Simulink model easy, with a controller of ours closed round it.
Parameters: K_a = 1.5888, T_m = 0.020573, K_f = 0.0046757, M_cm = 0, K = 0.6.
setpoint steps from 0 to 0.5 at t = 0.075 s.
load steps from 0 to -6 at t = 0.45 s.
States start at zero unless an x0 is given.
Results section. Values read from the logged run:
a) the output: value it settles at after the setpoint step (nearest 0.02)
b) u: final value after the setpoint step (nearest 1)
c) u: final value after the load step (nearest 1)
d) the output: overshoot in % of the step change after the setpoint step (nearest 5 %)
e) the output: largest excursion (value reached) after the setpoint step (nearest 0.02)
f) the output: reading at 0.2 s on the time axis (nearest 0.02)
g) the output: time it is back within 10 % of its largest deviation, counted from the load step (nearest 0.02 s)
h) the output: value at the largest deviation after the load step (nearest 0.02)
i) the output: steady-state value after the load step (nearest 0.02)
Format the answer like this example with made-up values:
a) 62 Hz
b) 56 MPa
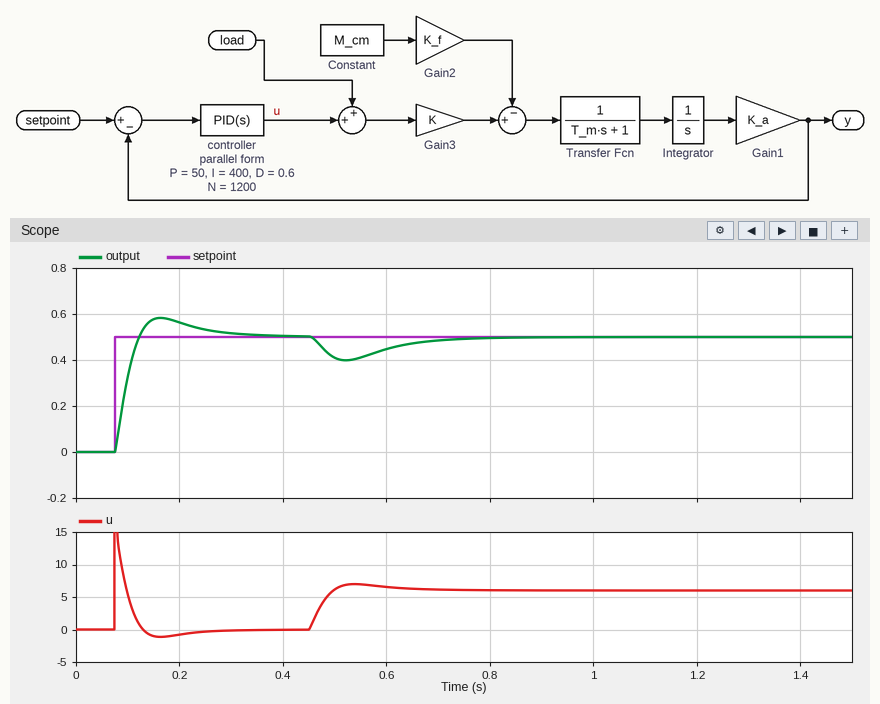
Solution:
a) 0.50
b) 0
c) 6
d) 15 %
e) 0.58
f) 0.56
g) 0.28 s
h) 0.40
i) 0.50
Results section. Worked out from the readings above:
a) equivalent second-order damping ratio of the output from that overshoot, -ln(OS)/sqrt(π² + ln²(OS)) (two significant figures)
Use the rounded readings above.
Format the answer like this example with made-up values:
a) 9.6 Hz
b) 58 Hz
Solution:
a) 0.52
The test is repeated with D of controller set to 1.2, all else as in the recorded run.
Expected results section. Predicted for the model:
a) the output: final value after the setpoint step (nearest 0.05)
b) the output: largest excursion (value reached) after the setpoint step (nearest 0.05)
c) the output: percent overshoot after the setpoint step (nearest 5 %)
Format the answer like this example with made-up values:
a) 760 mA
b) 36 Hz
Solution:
a) 0.50
b) 0.55
c) 10 %
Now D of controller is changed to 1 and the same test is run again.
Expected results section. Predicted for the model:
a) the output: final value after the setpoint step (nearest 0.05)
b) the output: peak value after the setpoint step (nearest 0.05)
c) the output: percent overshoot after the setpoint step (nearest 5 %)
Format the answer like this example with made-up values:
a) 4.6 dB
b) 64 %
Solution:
a) 0.50
b) 0.55
c) 10 %
